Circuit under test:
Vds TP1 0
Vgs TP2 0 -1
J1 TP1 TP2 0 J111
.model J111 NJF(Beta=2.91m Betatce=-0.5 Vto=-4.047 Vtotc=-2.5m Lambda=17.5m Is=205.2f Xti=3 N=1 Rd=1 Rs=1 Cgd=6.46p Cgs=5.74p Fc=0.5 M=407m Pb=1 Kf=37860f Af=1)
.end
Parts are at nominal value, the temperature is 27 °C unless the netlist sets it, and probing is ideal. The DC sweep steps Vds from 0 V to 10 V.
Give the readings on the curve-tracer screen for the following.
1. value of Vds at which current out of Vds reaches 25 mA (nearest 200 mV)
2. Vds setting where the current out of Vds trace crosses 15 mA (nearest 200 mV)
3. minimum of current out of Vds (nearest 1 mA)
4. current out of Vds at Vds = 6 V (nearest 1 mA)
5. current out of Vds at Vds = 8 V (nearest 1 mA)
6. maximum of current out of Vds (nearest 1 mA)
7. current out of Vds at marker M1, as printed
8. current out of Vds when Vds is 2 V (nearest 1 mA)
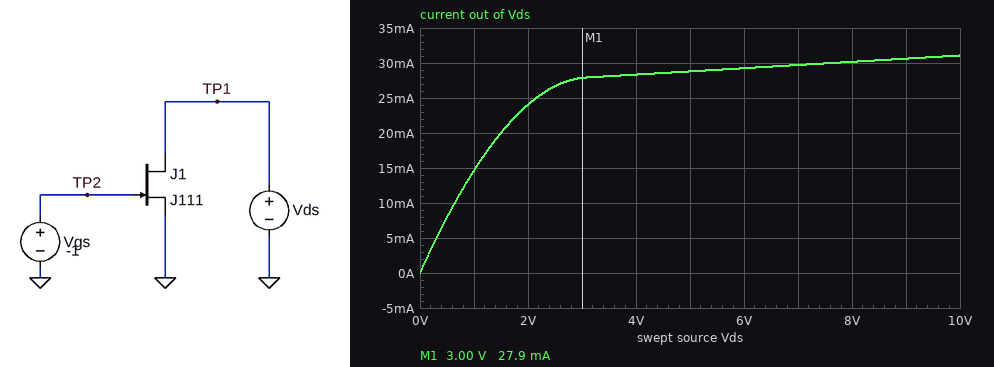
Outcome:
2.2 V
1.0 V
0 A
29 mA
30 mA
31 mA
27.9 mA
24 mA
